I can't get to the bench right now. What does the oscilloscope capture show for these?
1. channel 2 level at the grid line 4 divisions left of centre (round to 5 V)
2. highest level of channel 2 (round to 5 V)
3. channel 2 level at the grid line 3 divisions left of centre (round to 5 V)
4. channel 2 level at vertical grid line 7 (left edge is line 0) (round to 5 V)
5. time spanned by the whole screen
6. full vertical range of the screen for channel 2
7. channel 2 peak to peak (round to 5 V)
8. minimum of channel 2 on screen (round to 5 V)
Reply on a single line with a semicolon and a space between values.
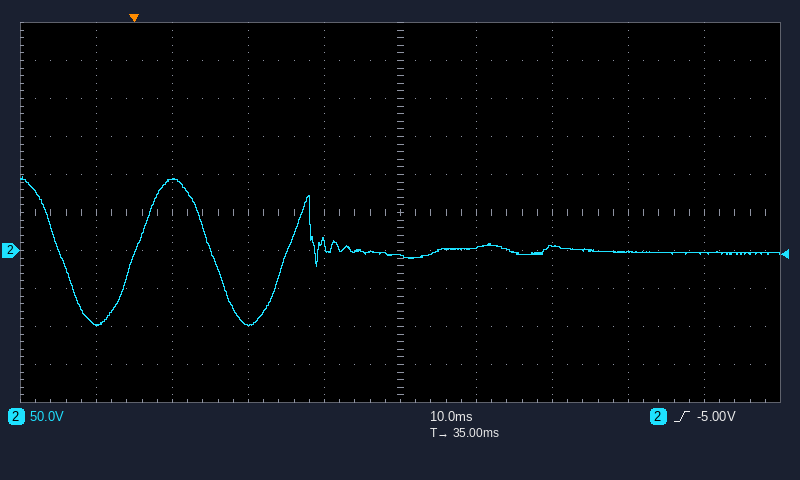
-95 V; 95 V; 95 V; 5 V; 100 ms; 500 V; 195 V; -100 V
